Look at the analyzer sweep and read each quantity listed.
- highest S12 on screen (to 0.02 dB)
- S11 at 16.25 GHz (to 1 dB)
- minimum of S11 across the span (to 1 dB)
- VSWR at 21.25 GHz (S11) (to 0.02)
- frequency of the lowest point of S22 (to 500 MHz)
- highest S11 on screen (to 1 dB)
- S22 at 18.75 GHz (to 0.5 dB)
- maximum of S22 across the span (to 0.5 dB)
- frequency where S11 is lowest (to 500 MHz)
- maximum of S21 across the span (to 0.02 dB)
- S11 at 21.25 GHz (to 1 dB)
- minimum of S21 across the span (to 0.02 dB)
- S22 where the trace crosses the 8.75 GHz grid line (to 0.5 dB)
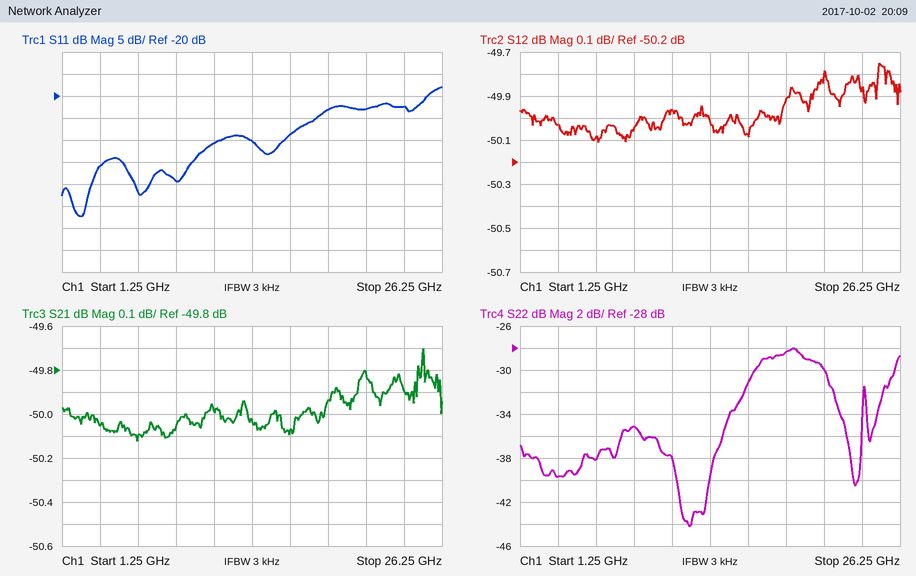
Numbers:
-49.76 dB
-29 dB
-47 dB
1.16
12.5 GHz
-18 dB
-28.5 dB
-28.0 dB
2.5 GHz
-49.70 dB
-23 dB
-50.12 dB
-35.0 dB
